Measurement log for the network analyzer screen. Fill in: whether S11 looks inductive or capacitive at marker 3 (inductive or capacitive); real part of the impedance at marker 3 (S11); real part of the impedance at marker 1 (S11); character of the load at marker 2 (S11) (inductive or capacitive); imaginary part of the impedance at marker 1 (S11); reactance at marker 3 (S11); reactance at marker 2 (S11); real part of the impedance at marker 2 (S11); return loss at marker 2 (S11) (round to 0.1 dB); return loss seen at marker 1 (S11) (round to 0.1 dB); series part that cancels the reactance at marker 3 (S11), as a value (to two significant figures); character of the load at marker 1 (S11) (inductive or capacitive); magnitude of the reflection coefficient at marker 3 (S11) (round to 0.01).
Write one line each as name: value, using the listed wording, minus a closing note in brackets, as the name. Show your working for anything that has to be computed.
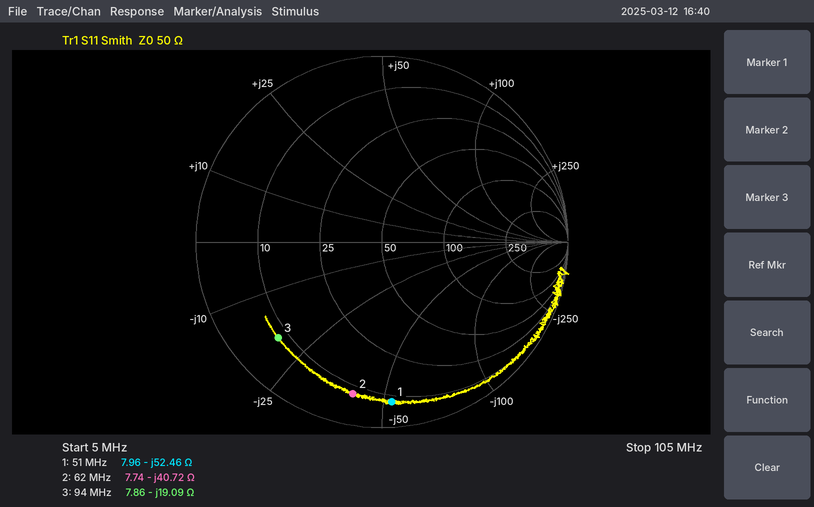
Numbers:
whether S11 looks inductive or capacitive at marker 3: capacitive
real part of the impedance at marker 3: 7.86 Ω
real part of the impedance at marker 1: 7.96 Ω
character of the load at marker 2 (S11): capacitive
imaginary part of the impedance at marker 1: -52.46 Ω
reactance at marker 3: -19.09 Ω
reactance at marker 2: -40.72 Ω
real part of the impedance at marker 2: 7.74 Ω
return loss at marker 2 (S11): 1.6 dB
return loss seen at marker 1 (S11): 1.3 dB
series part that cancels the reactance at marker 3 (S11), as a value: L = 19.09 Ω/(2π × 94 MHz) ≈ 32 nH
character of the load at marker 1 (S11): capacitive
magnitude of the reflection coefficient at marker 3 (S11): 0.76
